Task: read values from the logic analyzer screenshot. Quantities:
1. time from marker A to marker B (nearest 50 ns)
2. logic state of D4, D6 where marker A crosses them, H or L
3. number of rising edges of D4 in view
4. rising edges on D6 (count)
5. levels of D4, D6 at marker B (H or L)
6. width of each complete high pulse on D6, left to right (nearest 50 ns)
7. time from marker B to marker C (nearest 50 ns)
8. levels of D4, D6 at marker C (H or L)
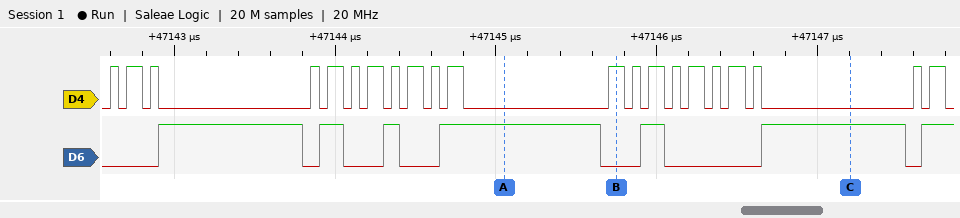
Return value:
700 ns
D4=L, D6=H
21
7
D4=H, D6=L
900 ns, 150 ns, 100 ns, 1000 ns, 150 ns, 900 ns
1450 ns
D4=L, D6=H
